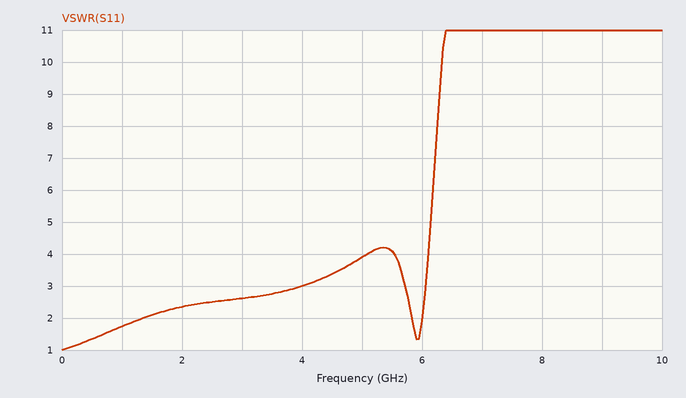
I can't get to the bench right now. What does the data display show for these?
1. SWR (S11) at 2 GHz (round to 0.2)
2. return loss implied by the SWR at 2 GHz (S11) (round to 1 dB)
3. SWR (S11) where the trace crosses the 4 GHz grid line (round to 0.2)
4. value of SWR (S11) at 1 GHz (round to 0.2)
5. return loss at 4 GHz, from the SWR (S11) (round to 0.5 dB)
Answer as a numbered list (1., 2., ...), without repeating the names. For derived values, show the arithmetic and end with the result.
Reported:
1. 2.4
2. −20 log10((2.4 − 1)/(2.4 + 1)) ≈ 8 dB
3. 3.0
4. 1.8
5. −20 log10((3 − 1)/(3 + 1)) ≈ 6.0 dB
